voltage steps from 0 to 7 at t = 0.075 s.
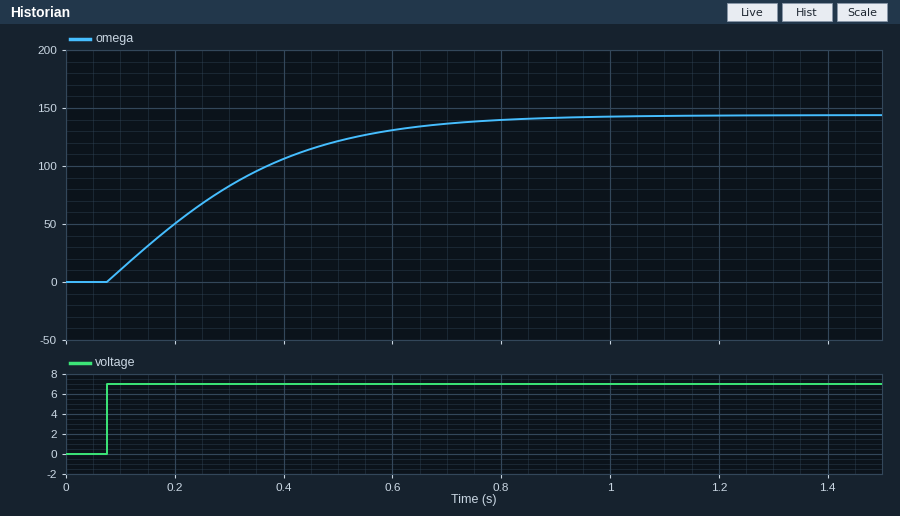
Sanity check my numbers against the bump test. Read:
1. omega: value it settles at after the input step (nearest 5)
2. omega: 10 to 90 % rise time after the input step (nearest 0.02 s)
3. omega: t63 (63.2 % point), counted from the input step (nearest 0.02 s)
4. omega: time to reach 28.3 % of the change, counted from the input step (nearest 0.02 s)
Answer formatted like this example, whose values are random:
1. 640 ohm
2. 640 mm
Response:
1. 145
2. 0.48 s
3. 0.26 s
4. 0.10 s
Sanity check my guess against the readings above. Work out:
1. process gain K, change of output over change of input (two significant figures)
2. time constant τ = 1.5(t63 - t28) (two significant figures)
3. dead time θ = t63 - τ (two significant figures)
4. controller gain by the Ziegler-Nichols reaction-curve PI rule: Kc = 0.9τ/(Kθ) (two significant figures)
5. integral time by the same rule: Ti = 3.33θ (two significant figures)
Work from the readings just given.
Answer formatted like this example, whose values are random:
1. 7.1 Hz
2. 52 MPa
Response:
1. 21
2. 0.24 s
3. 0.020 s
4. 0.51
5. 0.067 s
